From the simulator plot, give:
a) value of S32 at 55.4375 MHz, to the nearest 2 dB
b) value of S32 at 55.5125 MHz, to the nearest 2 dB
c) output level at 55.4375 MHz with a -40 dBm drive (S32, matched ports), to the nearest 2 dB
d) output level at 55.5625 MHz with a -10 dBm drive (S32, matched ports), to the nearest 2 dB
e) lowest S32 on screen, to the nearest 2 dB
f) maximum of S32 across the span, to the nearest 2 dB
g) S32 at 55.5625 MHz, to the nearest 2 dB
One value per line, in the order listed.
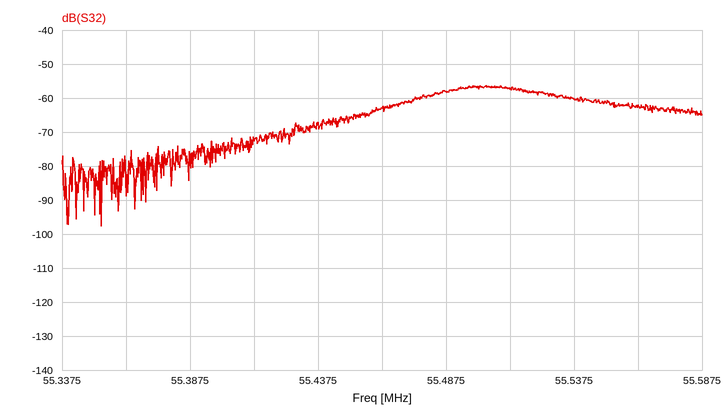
-68 dB
-58 dB
-108 dBm
-72 dBm
-98 dB
-56 dB
-62 dB
